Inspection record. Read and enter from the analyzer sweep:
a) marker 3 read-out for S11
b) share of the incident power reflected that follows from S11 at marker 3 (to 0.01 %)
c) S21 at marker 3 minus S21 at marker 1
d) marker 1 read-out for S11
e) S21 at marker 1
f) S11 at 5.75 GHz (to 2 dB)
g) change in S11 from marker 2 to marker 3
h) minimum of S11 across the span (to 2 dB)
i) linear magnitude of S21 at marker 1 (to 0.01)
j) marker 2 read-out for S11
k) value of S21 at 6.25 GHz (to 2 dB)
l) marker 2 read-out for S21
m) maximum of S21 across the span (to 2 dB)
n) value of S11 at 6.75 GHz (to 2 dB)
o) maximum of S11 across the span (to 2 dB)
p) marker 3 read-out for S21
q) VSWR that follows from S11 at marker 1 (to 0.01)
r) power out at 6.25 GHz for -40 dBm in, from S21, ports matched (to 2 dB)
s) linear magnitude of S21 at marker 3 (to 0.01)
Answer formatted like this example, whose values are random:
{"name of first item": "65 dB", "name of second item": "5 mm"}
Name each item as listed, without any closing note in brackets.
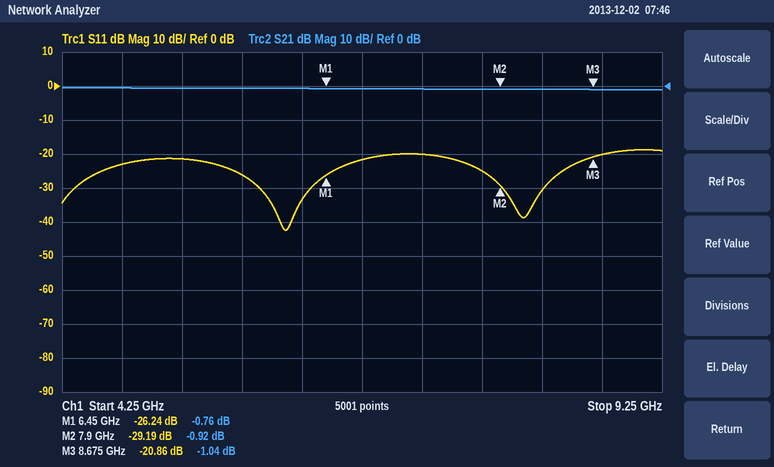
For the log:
{"marker 3 read-out for S11": "-20.86 dB", "share of the incident power reflected that follows from S11 at marker 3": "0.82 %", "S21 at marker 3 minus S21 at marker 1": "-0.28 dB", "marker 1 read-out for S11": "-26.24 dB", "S21 at marker 1": "-0.76 dB", "S11 at 5.75 GHz": "-26 dB", "change in S11 from marker 2 to marker 3": "8.33 dB", "minimum of S11 across the span": "-42 dB", "linear magnitude of S21 at marker 1": "0.92", "marker 2 read-out for S11": "-29.19 dB", "value of S21 at 6.25 GHz": "0 dB", "marker 2 read-out for S21": "-0.92 dB", "maximum of S21 across the span": "0 dB", "value of S11 at 6.75 GHz": "-22 dB", "maximum of S11 across the span": "-18 dB", "marker 3 read-out for S21": "-1.04 dB", "VSWR that follows from S11 at marker 1": "1.10", "power out at 6.25 GHz for -40 dBm in, from S21, ports matched": "-40 dBm", "linear magnitude of S21 at marker 3": "0.89"}
